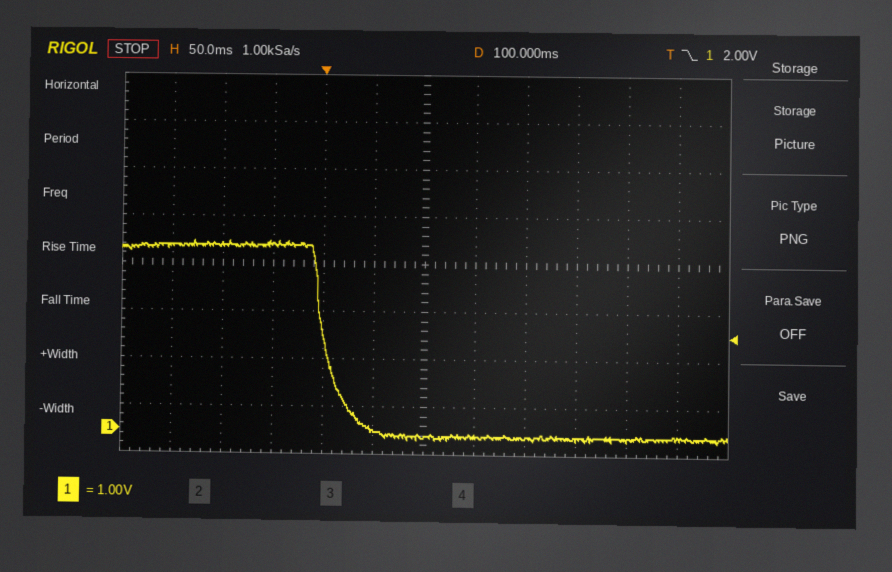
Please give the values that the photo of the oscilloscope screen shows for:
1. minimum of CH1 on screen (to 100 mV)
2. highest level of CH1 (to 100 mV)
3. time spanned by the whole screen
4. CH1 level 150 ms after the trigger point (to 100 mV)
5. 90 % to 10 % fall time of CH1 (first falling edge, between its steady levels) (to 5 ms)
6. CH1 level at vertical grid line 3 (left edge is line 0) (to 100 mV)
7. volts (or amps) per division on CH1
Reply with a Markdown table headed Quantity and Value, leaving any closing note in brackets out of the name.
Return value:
| Quantity | Value |
|---|---|
| minimum of CH1 on screen | -200 mV |
| highest level of CH1 | 4.0 V |
| time spanned by the whole screen | 600 ms |
| CH1 level 150 ms after the trigger point | -100 mV |
| 90 % to 10 % fall time of CH1 (first falling edge, between its steady levels) | 40 ms |
| CH1 level at vertical grid line 3 (left edge is line 0) | 3.9 V |
| volts (or amps) per division on CH1 | 1 V |
